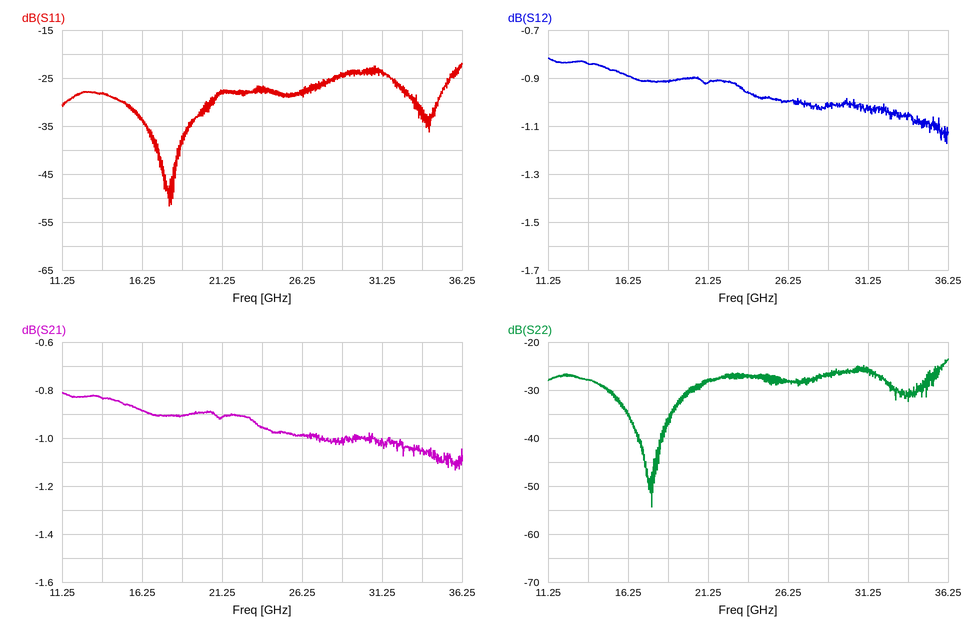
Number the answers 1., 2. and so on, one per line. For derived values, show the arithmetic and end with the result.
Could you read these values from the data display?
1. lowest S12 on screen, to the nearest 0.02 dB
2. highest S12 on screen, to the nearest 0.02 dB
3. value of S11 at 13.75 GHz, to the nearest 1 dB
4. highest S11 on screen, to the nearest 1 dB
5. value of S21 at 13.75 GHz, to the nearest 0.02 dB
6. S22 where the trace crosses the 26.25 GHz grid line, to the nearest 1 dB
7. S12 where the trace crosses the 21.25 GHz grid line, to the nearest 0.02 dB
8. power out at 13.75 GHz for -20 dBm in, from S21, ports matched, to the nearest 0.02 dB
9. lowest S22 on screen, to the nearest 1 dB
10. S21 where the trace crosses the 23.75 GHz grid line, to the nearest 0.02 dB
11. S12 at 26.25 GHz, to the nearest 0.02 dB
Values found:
1. -1.18 dB
2. -0.82 dB
3. -28 dB
4. -22 dB
5. -0.84 dB
6. -28 dB
7. -0.92 dB
8. -20 dBm + (-0.84 dB) = -20.84 dBm
9. -54 dB
10. -0.96 dB
11. -1.00 dB
